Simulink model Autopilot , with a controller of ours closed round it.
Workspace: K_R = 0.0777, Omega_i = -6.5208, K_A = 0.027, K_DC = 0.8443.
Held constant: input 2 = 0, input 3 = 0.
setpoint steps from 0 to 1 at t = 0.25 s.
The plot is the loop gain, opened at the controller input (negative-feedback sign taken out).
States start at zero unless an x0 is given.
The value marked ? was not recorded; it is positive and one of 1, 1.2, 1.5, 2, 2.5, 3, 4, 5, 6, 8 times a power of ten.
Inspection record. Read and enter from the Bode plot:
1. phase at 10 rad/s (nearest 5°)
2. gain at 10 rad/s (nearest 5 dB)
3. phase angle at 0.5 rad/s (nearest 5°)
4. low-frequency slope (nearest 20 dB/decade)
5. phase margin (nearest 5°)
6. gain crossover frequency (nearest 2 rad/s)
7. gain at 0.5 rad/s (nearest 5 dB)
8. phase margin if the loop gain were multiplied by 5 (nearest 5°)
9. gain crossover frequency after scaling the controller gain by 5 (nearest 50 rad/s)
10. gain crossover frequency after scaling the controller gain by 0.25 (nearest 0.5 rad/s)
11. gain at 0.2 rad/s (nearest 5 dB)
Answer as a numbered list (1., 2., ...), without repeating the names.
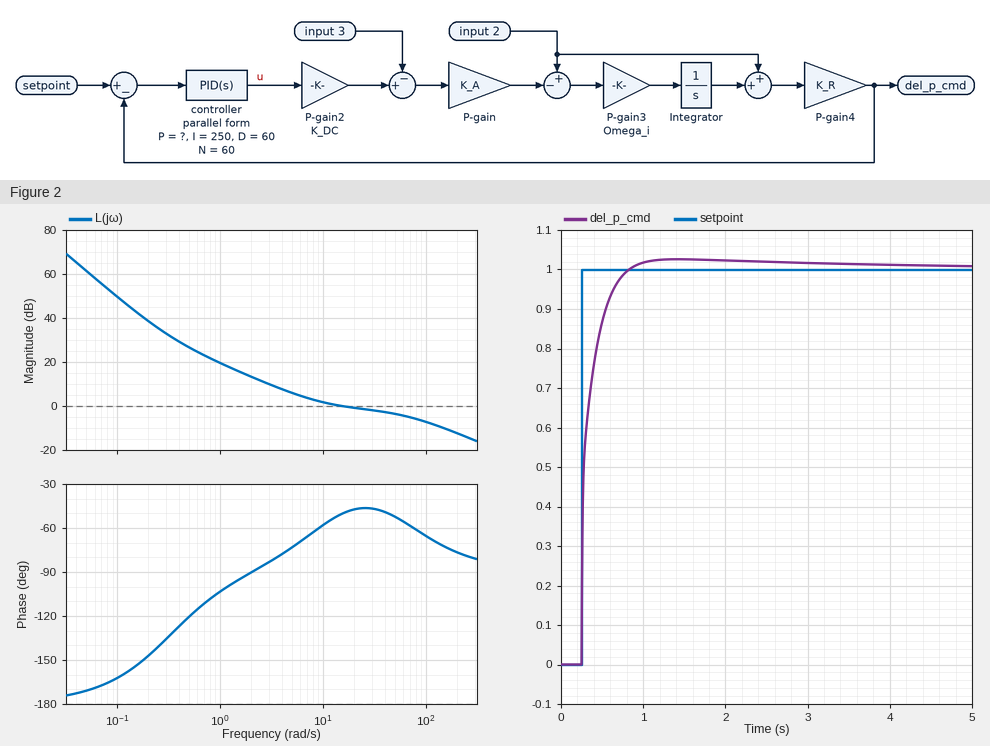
1. -60°
2. 0 dB
3. -120°
4. -40 dB/decade
5. 130°
6. 16 rad/s
7. 25 dB
8. 100°
9. 250 rad/s
10. 2.5 rad/s
11. 40 dB
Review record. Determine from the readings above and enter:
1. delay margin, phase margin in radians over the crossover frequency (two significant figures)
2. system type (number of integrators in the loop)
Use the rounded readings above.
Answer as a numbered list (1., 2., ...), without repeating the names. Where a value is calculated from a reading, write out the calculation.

1. 130 × π / 180 / 16 = 0.14 s
2. 2
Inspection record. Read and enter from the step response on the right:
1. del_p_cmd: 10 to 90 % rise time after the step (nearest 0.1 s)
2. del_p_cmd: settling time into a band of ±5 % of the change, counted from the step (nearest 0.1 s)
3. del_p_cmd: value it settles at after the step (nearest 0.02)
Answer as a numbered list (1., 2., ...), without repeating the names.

1. 0.3 s
2. 0.4 s
3. 1.00
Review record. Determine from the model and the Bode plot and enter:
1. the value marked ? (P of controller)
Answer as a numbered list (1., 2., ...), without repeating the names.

1. 800
